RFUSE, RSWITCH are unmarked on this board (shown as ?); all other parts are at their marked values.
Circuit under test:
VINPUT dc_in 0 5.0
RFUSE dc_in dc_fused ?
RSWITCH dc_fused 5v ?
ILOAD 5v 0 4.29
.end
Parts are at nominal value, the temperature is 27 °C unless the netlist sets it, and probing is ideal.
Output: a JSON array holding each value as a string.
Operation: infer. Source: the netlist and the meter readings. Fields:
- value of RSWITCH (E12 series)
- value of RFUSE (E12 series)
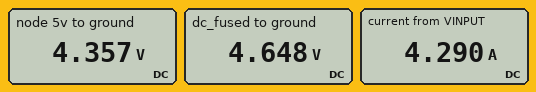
["0.068 Ω", "0.082 Ω"]
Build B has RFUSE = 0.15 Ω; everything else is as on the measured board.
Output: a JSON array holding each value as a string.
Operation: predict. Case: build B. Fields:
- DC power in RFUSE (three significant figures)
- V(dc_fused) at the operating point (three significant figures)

["2.76 W", "4.36 V"]
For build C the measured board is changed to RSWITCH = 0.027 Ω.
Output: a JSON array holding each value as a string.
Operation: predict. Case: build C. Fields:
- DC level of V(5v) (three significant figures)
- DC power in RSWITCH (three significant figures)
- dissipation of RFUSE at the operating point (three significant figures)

["4.53 V", "497 mW", "1.51 W"]
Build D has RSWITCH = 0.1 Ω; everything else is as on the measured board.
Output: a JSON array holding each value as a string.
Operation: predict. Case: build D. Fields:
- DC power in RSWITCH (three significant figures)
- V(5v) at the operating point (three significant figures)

["1.84 W", "4.22 V"]
